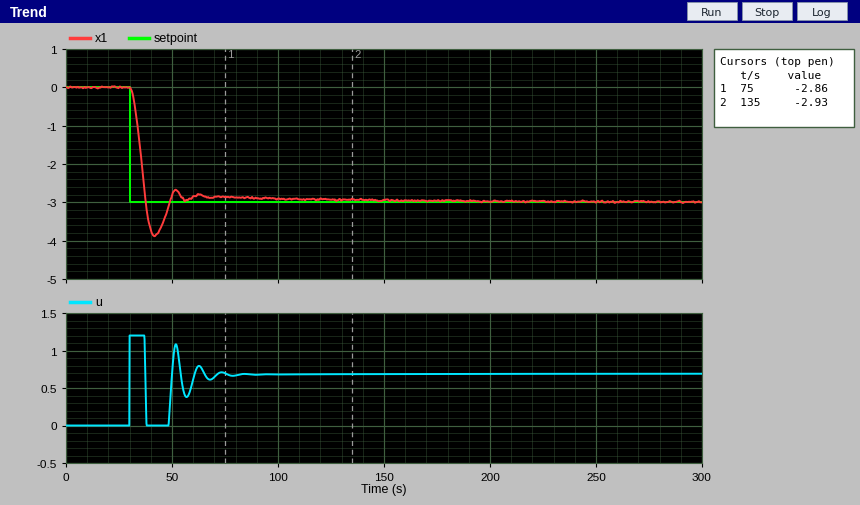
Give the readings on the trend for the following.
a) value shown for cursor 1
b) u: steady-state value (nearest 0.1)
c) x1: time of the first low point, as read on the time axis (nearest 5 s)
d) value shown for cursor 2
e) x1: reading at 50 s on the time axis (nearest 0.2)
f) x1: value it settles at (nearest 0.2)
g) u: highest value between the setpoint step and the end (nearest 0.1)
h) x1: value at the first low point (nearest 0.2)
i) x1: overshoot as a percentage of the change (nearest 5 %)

-2.86
0.7
40 s
-2.93
-2.8
-3.0
1.2
-3.8
30 %
